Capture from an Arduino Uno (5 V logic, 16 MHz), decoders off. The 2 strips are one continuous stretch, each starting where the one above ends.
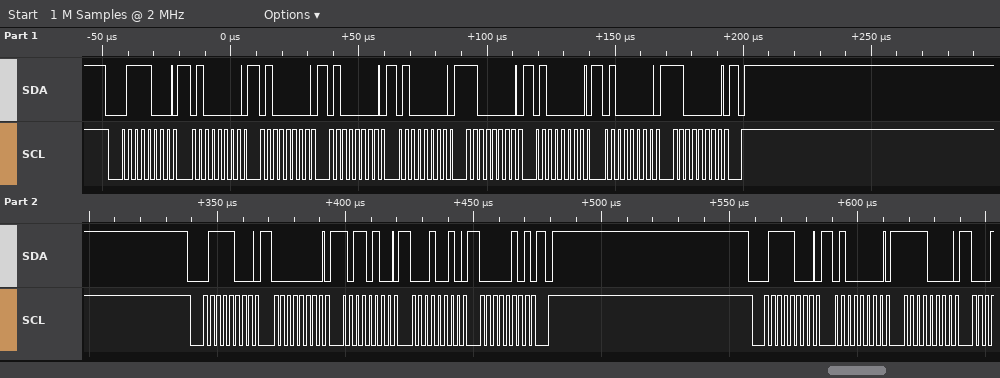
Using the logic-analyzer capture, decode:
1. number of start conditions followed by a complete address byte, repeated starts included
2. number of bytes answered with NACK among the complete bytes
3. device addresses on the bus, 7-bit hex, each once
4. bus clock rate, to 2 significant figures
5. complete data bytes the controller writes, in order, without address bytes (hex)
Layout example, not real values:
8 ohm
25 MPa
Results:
3
0
0x3C
400 kHz
40 40 40 40 C0 40 40 C0 00 B4 12 05 40 F0
